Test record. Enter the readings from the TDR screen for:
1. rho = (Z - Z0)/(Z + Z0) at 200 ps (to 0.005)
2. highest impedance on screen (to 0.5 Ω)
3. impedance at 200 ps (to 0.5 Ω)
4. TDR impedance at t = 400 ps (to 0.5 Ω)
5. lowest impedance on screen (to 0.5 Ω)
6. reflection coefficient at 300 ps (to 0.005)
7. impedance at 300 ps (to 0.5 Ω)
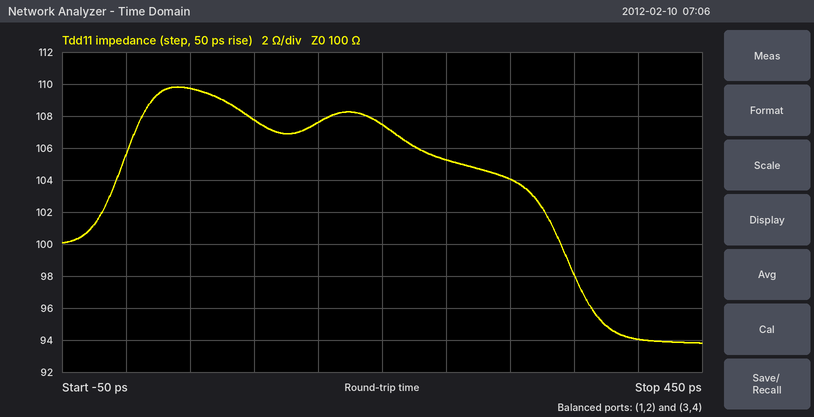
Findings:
+0.035
110.0 Ω
107.5 Ω
94.0 Ω
94.0 Ω
+0.020
104.0 Ω
